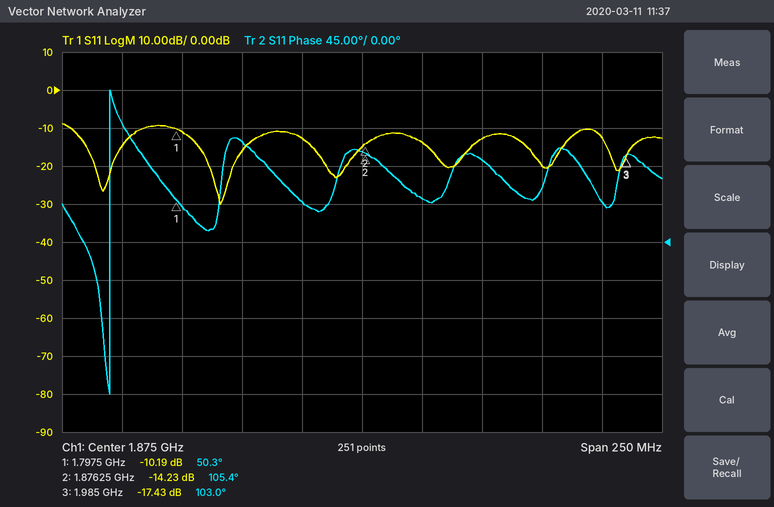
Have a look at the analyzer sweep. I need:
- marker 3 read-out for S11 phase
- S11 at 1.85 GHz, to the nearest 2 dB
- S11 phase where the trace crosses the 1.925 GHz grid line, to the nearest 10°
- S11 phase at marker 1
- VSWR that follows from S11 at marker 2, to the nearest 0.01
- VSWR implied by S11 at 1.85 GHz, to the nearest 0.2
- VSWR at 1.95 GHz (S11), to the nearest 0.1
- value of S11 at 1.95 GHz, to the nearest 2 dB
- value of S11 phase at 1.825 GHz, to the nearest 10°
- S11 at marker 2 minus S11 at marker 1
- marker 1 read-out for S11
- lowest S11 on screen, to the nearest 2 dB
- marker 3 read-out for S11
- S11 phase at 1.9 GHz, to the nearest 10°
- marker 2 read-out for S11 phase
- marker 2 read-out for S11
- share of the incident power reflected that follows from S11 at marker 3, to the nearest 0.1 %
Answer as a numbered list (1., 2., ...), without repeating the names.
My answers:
1. 103.0°
2. -12 dB
3. 100°
4. 50.3°
5. 1.48
6. 1.6
7. 1.2
8. -20 dB
9. 120°
10. -4.04 dB
11. -10.19 dB
12. -30 dB
13. -17.43 dB
14. 50°
15. 105.4°
16. -14.23 dB
17. 1.8 %
